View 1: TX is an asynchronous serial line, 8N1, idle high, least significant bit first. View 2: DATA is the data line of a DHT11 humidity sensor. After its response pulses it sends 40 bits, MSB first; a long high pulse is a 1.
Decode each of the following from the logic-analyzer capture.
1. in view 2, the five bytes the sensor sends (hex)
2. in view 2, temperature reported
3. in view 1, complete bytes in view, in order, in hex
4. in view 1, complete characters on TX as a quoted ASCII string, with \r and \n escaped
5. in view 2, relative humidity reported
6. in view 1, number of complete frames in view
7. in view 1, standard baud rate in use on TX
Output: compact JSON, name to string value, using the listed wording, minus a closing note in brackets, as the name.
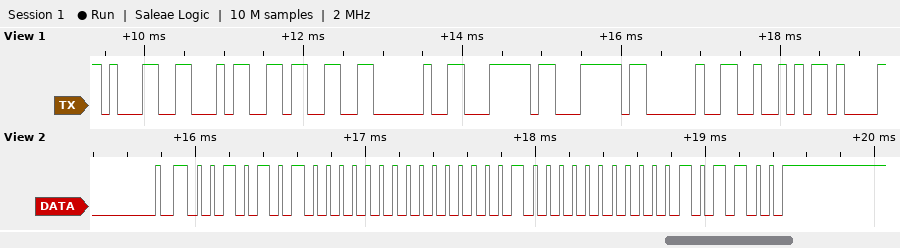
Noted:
{"in view 2, the five bytes the sensor sends": "2A 00 02 00 2C", "in view 2, temperature reported": "2.0 °C", "in view 1, complete bytes in view, in order, in hex": "0x31 0x34 0x33 0x20 0x7C 0x7C 0x20 0x52", "in view 1, complete characters on TX as a quoted ASCII string, with \\r and \\n escaped": "\"143 || R\"", "in view 2, relative humidity reported": "42 %", "in view 1, number of complete frames in view": "8", "in view 1, standard baud rate in use on TX": "9600 baud"}
